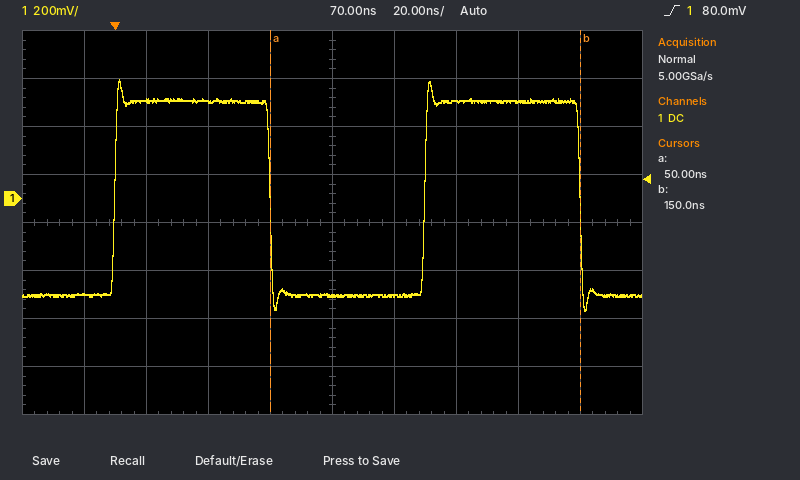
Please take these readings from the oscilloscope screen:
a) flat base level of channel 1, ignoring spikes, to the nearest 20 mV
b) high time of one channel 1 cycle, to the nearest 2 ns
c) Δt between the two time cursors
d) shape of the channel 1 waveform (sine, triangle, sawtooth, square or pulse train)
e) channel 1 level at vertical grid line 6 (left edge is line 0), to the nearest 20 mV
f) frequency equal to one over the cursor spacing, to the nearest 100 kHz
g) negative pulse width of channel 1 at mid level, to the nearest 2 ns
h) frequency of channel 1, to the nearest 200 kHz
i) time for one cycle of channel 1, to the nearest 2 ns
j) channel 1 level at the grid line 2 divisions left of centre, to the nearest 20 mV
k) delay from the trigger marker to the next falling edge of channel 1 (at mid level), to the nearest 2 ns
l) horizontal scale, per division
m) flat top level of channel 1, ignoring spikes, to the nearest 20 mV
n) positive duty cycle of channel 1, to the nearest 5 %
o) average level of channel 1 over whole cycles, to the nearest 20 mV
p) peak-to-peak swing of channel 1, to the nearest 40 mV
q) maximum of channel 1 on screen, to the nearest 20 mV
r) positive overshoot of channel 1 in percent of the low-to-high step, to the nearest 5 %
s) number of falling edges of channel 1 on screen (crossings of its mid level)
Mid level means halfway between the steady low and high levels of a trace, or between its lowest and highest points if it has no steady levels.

-400 mV
50 ns
100 ns
square
-400 mV
10.0 MHz
50 ns
10.0 MHz
100 ns
400 mV
50 ns
20 ns
400 mV
50 %
0 mV
960 mV
500 mV
10 %
2
